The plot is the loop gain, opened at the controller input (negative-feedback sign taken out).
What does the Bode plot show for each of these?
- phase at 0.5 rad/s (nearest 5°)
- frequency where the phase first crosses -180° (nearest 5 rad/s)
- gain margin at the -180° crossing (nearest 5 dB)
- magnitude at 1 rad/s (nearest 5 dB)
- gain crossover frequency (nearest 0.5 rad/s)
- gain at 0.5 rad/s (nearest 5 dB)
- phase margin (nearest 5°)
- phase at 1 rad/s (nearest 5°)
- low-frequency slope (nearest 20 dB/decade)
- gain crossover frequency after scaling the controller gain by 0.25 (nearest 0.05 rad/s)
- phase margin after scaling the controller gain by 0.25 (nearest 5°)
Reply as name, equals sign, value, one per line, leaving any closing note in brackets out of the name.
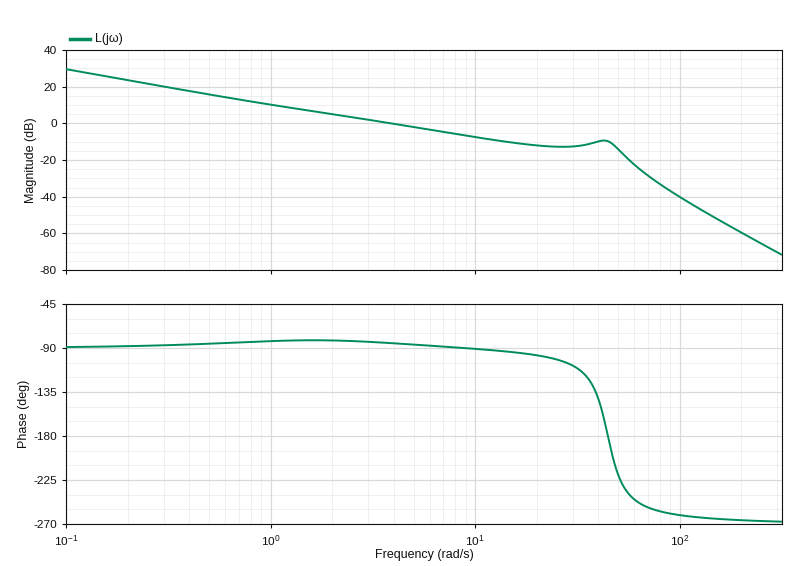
phase at 0.5 rad/s = -85°
frequency where the phase first crosses -180° = 45 rad/s
gain margin at the -180° crossing = 10 dB
magnitude at 1 rad/s = 10 dB
gain crossover frequency = 4.0 rad/s
gain at 0.5 rad/s = 15 dB
phase margin = 95°
phase at 1 rad/s = -85°
low-frequency slope = -20 dB/decade
gain crossover frequency after scaling the controller gain by 0.25 = 0.80 rad/s
phase margin after scaling the controller gain by 0.25 = 95°
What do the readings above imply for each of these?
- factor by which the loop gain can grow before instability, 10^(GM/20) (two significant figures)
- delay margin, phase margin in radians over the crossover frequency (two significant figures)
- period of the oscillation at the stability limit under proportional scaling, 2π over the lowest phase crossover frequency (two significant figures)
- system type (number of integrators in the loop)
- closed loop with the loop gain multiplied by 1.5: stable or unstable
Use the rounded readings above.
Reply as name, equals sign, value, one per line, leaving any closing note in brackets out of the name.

factor by which the loop gain can grow before instability, 10^(GM/20) = 3.2
delay margin, phase margin in radians over the crossover frequency = 0.41 s
period of the oscillation at the stability limit under proportional scaling, 2π over the lowest phase crossover frequency = 0.14 s
system type = 1
closed loop with the loop gain multiplied by 1.5: stable or unstable = stable
